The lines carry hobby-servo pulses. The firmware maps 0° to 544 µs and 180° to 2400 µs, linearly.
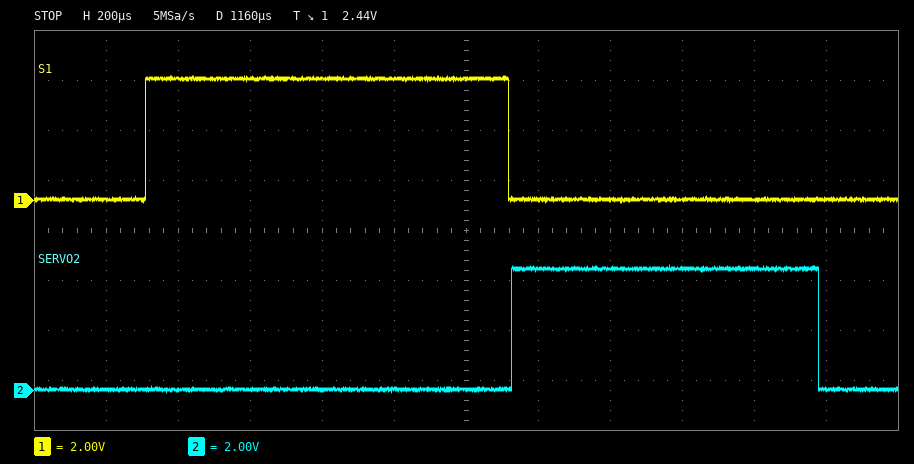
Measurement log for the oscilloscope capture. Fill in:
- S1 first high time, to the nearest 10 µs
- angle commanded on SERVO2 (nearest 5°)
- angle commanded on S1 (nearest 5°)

1010 µs
30°
45°
